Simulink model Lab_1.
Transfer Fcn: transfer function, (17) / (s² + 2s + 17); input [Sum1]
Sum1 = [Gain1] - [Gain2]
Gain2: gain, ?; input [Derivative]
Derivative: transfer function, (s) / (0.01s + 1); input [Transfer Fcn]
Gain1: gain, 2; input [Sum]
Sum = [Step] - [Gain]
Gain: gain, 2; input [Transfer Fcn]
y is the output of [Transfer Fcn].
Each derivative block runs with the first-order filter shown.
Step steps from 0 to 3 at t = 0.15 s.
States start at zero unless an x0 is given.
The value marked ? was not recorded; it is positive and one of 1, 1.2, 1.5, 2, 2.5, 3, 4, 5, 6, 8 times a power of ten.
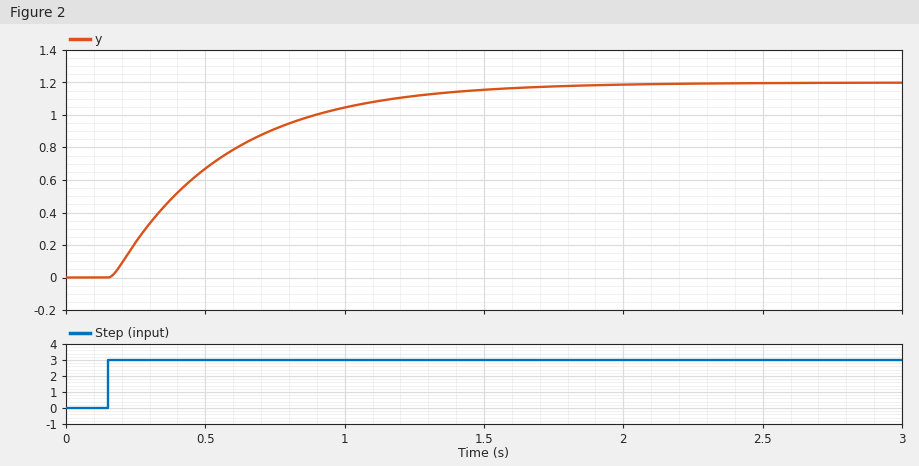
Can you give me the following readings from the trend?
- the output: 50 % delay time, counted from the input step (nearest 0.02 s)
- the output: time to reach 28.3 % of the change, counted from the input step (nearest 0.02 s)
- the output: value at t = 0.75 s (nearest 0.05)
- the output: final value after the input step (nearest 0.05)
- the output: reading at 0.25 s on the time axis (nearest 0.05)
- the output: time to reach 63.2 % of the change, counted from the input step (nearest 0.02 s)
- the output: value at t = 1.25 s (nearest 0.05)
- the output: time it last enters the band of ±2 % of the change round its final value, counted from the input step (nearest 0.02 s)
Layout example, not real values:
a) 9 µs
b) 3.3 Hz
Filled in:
a) 0.30 s
b) 0.16 s
c) 0.90
d) 1.20
e) 0.20
f) 0.42 s
g) 1.10
h) 1.60 s
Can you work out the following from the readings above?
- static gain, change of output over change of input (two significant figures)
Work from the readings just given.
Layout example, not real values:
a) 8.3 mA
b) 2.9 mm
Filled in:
a) 0.40
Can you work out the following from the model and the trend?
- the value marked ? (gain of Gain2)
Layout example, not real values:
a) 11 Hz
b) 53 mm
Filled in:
a) 2
